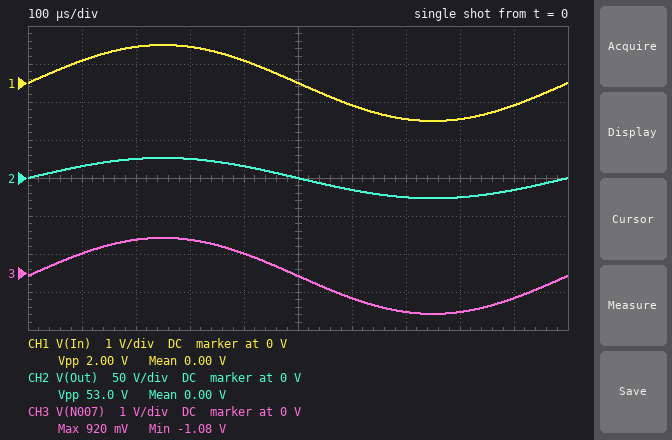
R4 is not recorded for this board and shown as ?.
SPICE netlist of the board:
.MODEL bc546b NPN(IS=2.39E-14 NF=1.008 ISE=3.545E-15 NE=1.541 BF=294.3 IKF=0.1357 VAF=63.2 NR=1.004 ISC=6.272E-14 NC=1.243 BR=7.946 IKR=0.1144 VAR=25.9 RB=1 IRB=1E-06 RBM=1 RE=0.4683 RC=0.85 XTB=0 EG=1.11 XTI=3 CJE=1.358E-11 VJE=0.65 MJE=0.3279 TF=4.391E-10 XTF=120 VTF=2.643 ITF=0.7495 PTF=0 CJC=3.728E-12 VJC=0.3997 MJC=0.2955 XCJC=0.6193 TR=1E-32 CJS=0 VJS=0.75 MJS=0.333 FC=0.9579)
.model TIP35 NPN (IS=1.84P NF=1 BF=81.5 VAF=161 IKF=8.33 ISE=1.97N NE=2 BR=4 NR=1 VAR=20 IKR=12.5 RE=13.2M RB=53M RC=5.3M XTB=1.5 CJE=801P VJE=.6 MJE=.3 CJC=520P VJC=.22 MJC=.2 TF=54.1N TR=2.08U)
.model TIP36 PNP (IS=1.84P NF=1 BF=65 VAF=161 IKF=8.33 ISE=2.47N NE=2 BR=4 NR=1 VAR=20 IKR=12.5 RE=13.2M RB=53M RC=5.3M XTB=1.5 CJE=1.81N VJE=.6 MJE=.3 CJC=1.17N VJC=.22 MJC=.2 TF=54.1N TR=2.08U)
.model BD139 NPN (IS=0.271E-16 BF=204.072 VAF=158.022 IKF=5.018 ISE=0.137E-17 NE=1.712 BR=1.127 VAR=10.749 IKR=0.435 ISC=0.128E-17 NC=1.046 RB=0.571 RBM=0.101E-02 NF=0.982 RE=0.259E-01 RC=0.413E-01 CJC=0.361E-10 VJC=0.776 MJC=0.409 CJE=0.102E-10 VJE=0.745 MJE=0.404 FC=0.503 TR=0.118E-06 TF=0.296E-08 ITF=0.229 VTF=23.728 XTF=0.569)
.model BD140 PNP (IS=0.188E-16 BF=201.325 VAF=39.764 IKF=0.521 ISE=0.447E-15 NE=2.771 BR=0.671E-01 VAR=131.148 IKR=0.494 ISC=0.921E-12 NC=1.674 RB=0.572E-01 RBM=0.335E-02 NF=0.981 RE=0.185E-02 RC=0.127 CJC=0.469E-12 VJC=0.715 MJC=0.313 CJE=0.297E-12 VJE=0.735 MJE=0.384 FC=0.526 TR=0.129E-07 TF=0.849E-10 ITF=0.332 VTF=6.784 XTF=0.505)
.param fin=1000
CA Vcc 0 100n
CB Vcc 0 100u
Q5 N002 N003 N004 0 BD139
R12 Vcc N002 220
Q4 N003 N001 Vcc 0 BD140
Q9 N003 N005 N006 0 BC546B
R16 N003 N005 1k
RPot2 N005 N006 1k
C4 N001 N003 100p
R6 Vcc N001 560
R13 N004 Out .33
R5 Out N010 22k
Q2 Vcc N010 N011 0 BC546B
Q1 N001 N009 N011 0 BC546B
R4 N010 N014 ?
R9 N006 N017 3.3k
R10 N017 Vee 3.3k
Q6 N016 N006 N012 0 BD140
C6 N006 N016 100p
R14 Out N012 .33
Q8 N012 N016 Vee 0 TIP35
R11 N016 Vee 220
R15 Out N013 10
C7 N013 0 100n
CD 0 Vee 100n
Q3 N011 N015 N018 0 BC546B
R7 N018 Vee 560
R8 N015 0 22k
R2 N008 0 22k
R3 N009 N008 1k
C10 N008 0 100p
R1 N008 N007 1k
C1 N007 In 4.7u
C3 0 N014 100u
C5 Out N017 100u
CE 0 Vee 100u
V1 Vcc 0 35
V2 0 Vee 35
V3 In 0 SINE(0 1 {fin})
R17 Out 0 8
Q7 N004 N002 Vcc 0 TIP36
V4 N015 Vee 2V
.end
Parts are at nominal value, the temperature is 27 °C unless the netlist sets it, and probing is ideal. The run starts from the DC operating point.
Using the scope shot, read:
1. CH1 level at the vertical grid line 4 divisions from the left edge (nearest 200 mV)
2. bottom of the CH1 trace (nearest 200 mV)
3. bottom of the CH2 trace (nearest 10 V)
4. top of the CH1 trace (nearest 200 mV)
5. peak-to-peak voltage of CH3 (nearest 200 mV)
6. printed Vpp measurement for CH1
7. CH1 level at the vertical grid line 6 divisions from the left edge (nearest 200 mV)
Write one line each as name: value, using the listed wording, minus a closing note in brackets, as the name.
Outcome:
CH1 level at the vertical grid line 4 divisions from the left edge: 600 mV
bottom of the CH1 trace: -1.0 V
bottom of the CH2 trace: -30 V
top of the CH1 trace: 1.0 V
peak-to-peak voltage of CH3: 2.0 V
printed Vpp measurement for CH1: 2.00 V
CH1 level at the vertical grid line 6 divisions from the left edge: -600 mV
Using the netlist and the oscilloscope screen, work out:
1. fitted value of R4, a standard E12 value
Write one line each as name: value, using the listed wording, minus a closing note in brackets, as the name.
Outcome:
fitted value of R4, a standard E12 value: 820 Ω
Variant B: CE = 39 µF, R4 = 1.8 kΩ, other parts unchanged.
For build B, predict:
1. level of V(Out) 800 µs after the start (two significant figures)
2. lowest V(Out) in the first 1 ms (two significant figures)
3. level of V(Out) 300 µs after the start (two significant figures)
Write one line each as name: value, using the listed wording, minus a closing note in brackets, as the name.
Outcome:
level of V(Out) 800 µs after the start: -12 V
lowest V(Out) in the first 1 ms: -13 V
level of V(Out) 300 µs after the start: 12 V
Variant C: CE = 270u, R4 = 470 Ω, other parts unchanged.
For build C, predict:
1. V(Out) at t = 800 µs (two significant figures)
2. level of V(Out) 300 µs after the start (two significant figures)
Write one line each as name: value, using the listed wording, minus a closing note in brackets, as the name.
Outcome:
V(Out) at t = 800 µs: -33 V
level of V(Out) 300 µs after the start: 33 V
